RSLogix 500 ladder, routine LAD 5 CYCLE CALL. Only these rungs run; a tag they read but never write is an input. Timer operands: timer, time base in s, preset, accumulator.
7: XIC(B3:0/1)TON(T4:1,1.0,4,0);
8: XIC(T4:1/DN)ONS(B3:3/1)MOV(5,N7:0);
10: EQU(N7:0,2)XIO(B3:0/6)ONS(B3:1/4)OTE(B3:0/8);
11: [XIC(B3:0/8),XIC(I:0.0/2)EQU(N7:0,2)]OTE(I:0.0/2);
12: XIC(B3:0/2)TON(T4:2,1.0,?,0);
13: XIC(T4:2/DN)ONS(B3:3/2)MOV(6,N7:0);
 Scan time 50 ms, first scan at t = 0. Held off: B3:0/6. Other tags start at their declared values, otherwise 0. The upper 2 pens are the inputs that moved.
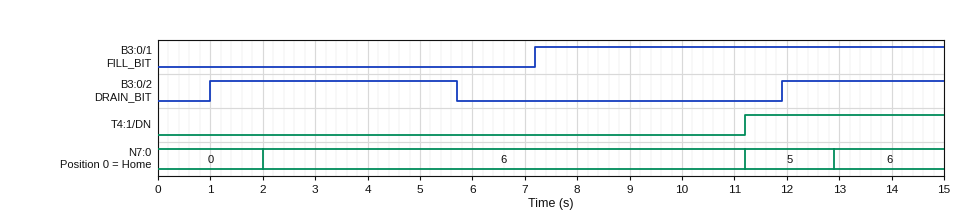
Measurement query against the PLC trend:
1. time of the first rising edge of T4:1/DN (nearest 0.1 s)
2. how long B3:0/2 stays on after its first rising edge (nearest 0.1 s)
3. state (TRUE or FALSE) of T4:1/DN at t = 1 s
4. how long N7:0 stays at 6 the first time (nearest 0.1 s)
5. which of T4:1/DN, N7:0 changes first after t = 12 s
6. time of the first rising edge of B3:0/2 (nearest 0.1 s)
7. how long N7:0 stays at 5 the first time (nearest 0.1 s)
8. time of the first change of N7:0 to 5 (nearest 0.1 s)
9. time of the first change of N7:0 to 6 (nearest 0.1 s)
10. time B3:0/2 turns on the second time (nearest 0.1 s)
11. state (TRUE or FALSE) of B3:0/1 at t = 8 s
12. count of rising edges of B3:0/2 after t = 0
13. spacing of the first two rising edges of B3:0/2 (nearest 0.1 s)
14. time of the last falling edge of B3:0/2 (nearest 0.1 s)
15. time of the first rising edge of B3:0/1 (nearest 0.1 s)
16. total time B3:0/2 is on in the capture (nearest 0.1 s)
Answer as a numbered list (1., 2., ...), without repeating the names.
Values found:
1. 11.2 s
2. 4.7 s
3. FALSE
4. 9.2 s
5. N7:0
6. 1.0 s
7. 1.7 s
8. 11.2 s
9. 2.0 s
10. 11.9 s
11. TRUE
12. 2
13. 10.9 s
14. 5.7 s
15. 7.2 s
16. 7.8 s
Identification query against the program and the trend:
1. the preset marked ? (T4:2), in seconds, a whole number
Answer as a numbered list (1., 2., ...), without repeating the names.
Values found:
1. 1 s
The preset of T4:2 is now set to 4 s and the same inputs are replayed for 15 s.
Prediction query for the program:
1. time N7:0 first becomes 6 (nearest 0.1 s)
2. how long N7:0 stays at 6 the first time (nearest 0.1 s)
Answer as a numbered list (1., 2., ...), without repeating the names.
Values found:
1. 5.0 s
2. 6.2 s
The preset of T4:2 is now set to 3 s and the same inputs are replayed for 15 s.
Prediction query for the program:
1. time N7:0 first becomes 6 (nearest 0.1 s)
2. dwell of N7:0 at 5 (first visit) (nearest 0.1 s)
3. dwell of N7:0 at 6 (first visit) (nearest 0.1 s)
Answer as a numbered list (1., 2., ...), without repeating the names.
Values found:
1. 4.0 s
2. 3.7 s
3. 7.2 s
